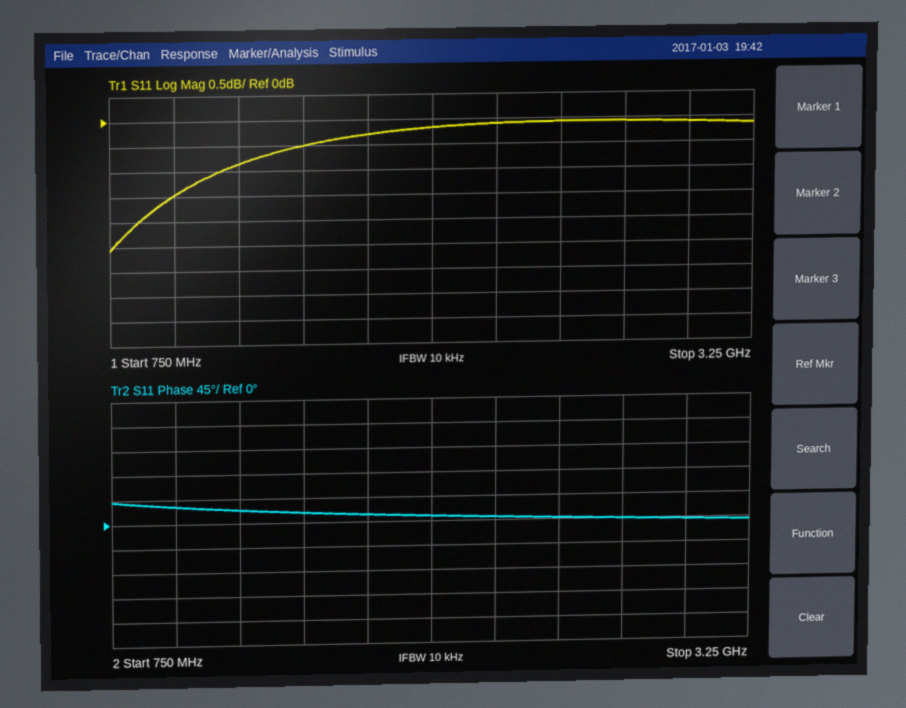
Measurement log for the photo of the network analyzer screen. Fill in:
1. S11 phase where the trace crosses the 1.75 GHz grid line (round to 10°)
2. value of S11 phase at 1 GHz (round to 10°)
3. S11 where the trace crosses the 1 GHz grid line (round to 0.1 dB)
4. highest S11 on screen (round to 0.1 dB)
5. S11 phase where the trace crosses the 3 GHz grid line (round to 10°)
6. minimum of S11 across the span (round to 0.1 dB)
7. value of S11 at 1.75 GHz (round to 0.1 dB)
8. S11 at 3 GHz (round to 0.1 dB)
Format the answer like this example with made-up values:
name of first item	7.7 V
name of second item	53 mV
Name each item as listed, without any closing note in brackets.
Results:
S11 phase where the trace crosses the 1.75 GHz grid line	10°
value of S11 phase at 1 GHz	30°
S11 where the trace crosses the 1 GHz grid line	-1.5 dB
highest S11 on screen	-0.1 dB
S11 phase where the trace crosses the 3 GHz grid line	0°
minimum of S11 across the span	-2.6 dB
value of S11 at 1.75 GHz	-0.3 dB
S11 at 3 GHz	-0.1 dB
